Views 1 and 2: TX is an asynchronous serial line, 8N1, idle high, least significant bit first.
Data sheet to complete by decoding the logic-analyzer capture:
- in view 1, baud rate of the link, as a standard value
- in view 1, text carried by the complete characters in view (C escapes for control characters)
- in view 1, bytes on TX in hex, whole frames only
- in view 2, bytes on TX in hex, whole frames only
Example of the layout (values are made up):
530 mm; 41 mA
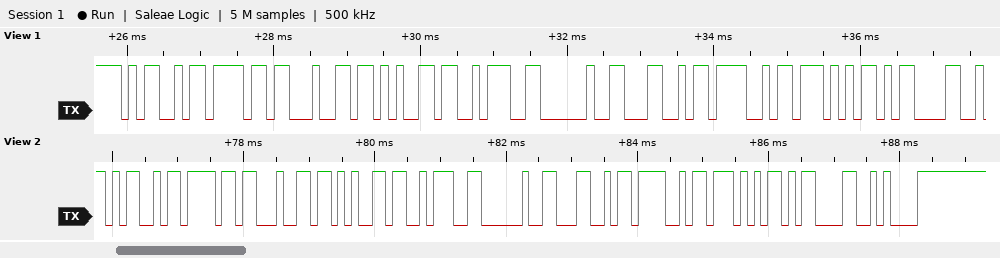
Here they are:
9600 baud; "Mode: LOW\r"; 4D 6F 64 65 3A 20 4C 4F 57 0D; 4D 6F 64 65 3A 20 4C 4F 57 0D 0A
